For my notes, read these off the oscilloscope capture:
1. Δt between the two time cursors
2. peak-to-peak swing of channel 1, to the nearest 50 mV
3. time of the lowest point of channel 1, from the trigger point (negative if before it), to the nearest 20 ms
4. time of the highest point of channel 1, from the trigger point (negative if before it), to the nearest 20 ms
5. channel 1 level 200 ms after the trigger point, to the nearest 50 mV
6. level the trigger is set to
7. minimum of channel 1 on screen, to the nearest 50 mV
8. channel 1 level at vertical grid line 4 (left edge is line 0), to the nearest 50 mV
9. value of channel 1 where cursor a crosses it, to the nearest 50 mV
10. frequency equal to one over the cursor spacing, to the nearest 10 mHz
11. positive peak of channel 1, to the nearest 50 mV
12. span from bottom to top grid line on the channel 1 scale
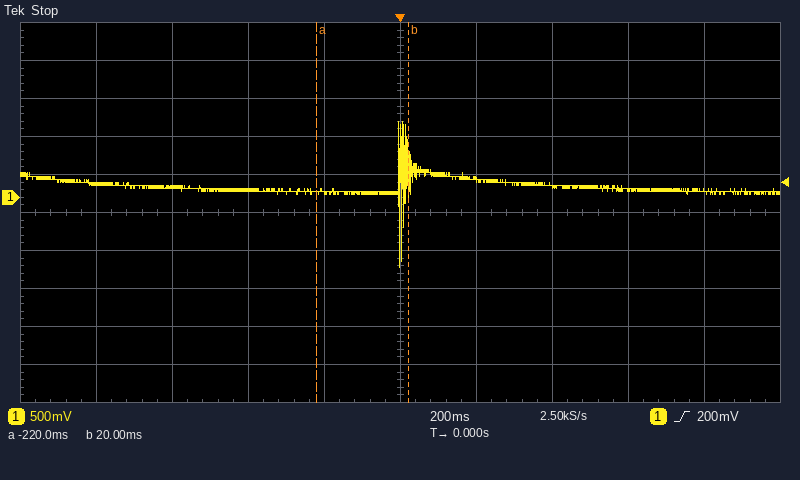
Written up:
240 ms
1.90 V
0 ms
0 ms
250 mV
200 mV
-900 mV
100 mV
50 mV
4.17 Hz
1.00 V
5 V
